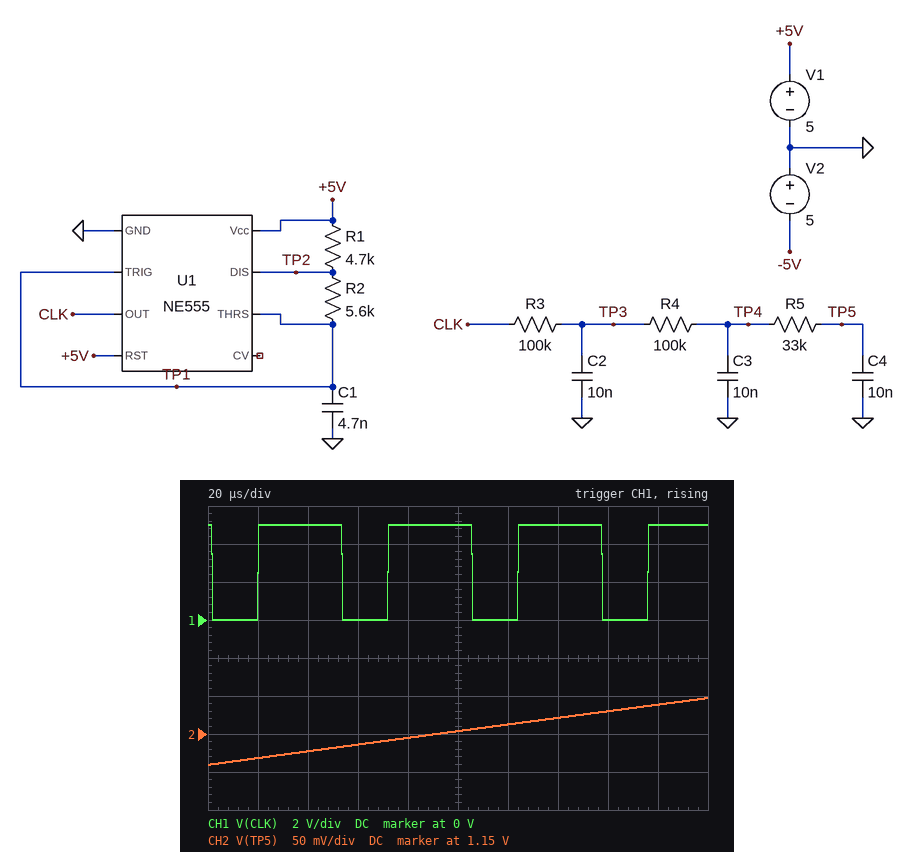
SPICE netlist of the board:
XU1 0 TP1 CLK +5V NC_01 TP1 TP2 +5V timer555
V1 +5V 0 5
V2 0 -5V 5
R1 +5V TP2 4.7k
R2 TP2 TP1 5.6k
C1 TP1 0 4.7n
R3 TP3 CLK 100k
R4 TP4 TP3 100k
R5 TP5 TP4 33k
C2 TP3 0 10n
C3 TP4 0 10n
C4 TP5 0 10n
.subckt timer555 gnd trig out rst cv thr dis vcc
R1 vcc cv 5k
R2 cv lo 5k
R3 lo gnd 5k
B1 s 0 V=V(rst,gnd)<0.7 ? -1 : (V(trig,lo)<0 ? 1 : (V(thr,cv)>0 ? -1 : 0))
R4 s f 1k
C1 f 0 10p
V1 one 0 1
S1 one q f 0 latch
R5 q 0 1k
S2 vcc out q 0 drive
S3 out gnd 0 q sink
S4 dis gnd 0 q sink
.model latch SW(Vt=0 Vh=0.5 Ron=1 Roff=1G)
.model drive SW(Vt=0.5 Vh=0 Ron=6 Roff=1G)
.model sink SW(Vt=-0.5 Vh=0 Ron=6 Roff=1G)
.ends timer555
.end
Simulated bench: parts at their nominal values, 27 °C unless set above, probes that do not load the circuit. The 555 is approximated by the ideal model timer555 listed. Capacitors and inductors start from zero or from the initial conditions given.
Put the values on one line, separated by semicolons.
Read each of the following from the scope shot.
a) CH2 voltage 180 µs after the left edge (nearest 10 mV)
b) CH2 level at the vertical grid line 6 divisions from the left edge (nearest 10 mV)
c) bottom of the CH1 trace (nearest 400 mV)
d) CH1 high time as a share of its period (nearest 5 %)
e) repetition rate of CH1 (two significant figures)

1.19 V; 1.16 V; 0 V; 65 %; 19 kHz
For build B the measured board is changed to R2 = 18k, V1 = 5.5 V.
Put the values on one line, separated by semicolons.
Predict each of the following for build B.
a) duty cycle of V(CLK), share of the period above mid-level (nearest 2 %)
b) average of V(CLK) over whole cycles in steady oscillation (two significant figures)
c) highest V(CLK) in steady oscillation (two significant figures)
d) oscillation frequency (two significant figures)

56 %; 3.1 V; 5.5 V; 7.5 kHz
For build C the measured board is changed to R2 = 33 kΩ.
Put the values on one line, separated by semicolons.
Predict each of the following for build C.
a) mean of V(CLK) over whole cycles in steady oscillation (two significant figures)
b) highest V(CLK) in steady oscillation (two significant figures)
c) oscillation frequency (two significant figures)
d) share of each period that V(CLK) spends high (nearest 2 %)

2.7 V; 5.0 V; 4.3 kHz; 54 %
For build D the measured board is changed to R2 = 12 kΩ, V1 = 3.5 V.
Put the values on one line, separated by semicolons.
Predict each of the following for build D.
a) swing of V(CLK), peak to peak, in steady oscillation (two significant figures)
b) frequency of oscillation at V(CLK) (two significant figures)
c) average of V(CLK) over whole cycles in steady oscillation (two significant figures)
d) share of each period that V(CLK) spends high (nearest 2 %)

3.5 V; 11 kHz; 2.0 V; 58 %
